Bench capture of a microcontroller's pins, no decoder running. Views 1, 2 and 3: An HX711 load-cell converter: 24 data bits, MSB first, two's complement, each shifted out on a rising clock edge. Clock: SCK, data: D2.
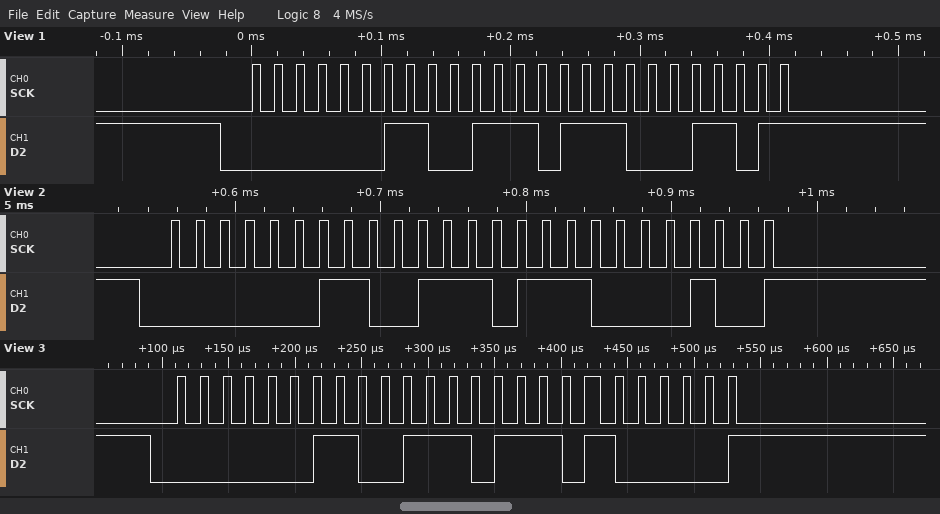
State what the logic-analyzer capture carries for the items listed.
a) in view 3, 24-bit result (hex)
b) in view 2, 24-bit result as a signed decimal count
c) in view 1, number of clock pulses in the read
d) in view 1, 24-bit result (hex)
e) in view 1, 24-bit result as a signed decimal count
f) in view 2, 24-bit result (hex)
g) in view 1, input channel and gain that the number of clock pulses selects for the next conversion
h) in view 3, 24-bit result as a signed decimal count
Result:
0x033BA0
211844
25
0x033B8D
211853
0x033B84
channel A, gain 128
211872
